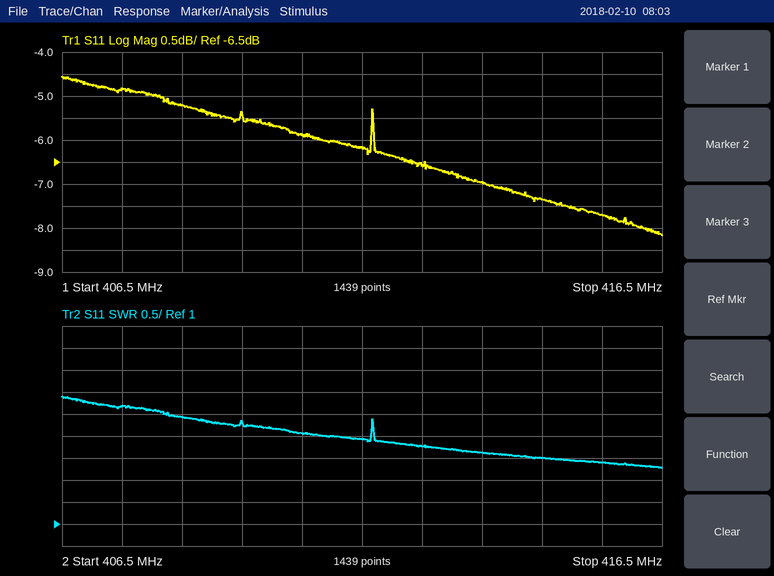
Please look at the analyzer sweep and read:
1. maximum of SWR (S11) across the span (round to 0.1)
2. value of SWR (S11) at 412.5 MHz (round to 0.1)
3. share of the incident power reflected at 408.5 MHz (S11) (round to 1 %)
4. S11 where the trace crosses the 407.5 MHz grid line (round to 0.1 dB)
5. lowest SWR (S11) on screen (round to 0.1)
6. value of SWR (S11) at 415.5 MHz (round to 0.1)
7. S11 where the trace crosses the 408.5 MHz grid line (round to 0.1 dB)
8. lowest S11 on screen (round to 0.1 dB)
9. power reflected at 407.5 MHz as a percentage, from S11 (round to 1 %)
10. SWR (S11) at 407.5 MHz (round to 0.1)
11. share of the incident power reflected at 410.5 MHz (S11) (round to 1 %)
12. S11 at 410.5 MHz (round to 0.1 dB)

3.9
2.8
30 %
-4.8 dB
2.3
2.4
-5.2 dB
-8.2 dB
33 %
3.7
26 %
-5.9 dB
